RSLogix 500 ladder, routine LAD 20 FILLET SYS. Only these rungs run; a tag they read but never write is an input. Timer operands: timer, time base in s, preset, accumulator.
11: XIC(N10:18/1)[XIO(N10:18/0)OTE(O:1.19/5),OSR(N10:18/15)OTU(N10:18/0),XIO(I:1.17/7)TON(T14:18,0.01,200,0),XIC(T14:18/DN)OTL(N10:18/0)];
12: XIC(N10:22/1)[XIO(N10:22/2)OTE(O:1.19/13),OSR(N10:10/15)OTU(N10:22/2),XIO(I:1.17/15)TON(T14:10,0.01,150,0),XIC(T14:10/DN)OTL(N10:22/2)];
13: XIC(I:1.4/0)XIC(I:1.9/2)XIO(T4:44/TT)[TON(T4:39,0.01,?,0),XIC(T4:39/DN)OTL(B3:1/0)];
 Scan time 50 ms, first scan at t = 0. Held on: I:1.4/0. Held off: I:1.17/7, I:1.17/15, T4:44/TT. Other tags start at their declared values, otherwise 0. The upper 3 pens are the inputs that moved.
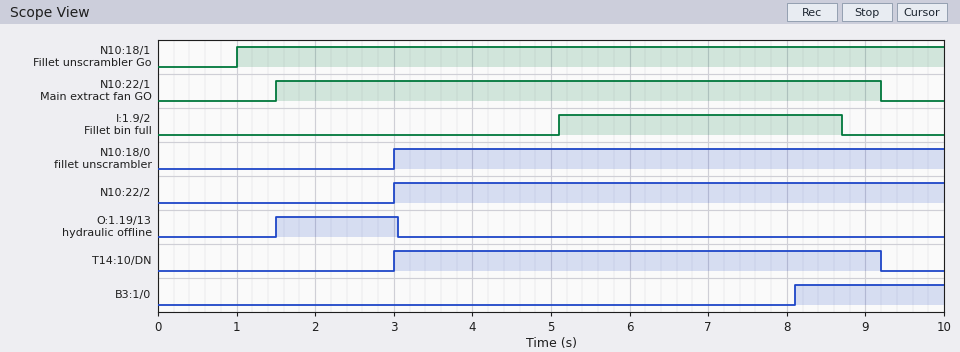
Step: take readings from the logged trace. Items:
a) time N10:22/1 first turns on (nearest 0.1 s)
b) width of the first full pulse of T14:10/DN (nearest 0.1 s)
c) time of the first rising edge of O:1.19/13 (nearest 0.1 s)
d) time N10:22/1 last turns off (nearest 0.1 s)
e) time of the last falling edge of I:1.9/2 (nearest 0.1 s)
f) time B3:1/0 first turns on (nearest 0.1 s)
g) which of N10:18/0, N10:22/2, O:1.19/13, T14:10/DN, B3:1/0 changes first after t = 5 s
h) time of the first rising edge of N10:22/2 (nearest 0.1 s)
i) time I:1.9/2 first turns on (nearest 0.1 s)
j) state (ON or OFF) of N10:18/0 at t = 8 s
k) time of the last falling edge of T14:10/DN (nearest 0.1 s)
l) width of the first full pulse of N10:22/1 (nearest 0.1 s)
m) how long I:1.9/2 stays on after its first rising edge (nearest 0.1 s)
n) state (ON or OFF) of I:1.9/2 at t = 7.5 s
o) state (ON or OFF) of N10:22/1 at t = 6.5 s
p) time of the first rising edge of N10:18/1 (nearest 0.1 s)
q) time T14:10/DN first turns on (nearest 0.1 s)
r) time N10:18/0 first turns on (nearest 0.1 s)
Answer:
1.5 s
6.2 s
1.5 s
9.2 s
8.7 s
8.1 s
B3:1/0
3.0 s
5.1 s
ON
9.2 s
7.7 s
3.6 s
ON
ON
1.0 s
3.0 s
3.0 s
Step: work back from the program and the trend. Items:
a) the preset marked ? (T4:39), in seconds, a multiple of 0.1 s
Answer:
3.0 s
